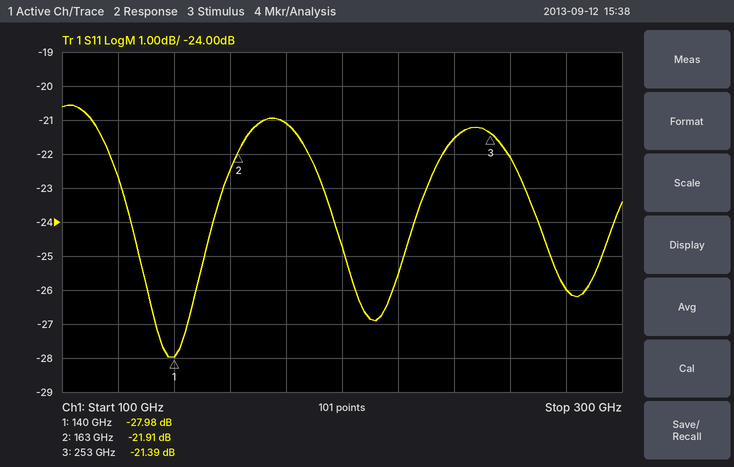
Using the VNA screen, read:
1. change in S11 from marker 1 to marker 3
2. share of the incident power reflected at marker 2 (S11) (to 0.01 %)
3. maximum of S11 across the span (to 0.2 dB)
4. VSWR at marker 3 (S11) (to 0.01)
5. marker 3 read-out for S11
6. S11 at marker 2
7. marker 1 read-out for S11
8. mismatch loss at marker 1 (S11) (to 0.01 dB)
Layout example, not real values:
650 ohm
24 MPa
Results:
6.59 dB
0.64 %
-20.6 dB
1.19
-21.39 dB
-21.91 dB
-27.98 dB
0.01 dB
